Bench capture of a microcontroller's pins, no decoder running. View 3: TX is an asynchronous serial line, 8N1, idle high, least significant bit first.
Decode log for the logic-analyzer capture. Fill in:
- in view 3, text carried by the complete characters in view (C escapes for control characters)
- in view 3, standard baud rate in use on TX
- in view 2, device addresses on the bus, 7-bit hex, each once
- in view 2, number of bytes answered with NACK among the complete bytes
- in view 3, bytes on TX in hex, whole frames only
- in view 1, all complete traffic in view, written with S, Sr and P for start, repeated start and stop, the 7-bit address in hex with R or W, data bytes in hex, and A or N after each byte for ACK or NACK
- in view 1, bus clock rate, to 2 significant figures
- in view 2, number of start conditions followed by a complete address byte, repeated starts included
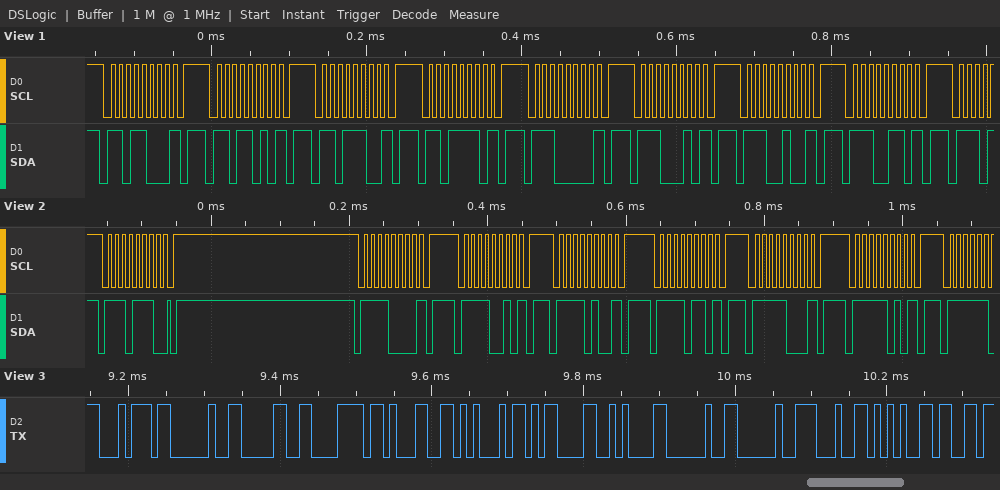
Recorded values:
"t 0x1E\r\n  de"
115200 baud
0x77 0x78 0x79 0x7A 0x7B 0x7C 0x7D
6
74 20 30 78 31 45 0D 0A 20 20 64 65
S 6CW N P S 6DW N P S 6EW N P S 6FW N P S 70W N P S 71W N P S 72W N P S 73W N P
100 kHz
7
